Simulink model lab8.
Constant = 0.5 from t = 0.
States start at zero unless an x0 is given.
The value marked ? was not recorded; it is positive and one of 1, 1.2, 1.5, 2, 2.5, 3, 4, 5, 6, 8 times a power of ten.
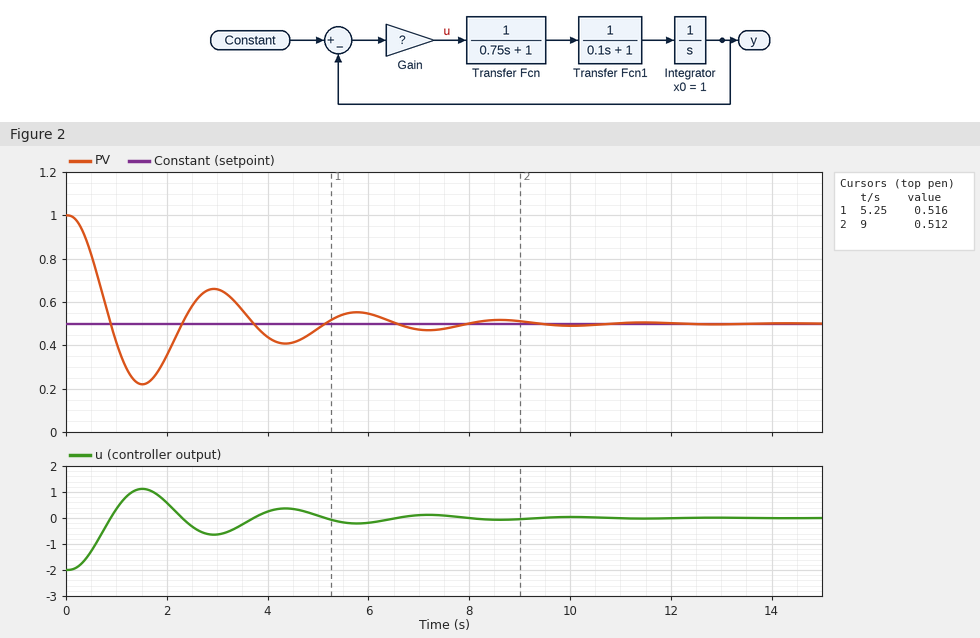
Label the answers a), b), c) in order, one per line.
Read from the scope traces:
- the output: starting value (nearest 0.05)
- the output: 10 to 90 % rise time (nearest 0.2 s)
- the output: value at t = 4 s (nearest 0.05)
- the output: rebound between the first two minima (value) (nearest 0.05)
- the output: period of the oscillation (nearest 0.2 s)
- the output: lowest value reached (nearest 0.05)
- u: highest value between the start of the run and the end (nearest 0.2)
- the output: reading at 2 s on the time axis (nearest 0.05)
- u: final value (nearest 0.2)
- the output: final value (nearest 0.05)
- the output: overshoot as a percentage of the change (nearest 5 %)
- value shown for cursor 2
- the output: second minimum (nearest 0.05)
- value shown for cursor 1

a) 1.00
b) 0.6 s
c) 0.45
d) 0.65
e) 2.8 s
f) 0.20
g) 1.2
h) 0.35
i) 0.0
j) 0.50
k) 55 %
l) 0.512
m) 0.40
n) 0.516
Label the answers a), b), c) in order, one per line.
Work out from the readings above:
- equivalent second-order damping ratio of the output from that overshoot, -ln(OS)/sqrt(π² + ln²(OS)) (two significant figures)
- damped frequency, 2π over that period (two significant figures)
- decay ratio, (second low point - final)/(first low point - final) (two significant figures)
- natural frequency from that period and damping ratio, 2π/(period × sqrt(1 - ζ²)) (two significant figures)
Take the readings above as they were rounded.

a) 0.19
b) 2.2 rad/s
c) 0.33
d) 2.3 rad/s
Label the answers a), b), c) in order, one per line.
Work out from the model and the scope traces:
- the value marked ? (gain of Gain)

a) 4
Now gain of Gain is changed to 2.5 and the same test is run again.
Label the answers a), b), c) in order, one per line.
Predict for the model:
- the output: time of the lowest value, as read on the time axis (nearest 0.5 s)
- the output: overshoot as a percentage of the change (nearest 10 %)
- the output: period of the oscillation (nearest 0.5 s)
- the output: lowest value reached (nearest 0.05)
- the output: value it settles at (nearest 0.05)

a) 2.0 s
b) 40 %
c) 3.5 s
d) 0.30
e) 0.50
